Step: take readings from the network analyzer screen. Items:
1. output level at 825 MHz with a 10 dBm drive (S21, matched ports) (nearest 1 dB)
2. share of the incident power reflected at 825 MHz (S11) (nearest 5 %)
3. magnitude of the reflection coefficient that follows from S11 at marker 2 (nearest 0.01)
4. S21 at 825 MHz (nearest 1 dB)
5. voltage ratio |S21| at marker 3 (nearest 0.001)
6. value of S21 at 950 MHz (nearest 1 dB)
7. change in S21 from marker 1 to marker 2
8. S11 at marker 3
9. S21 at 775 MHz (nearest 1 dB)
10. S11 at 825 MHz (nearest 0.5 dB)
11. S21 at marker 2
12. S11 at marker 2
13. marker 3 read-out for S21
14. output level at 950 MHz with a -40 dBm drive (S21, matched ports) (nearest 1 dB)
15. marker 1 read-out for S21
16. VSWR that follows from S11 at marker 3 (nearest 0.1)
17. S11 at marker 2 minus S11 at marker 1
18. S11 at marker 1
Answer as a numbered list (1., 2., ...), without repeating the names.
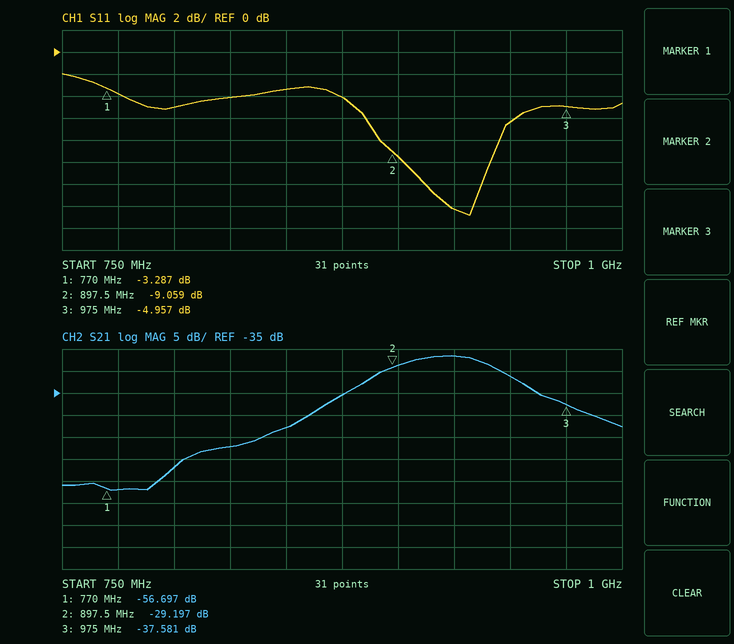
1. -37 dBm
2. 40 %
3. 0.35
4. -47 dB
5. 0.013
6. -31 dB
7. 27.500 dB
8. -4.957 dB
9. -57 dB
10. -4.0 dB
11. -29.197 dB
12. -9.059 dB
13. -37.581 dB
14. -71 dBm
15. -56.697 dB
16. 3.6
17. -5.772 dB
18. -3.287 dB
